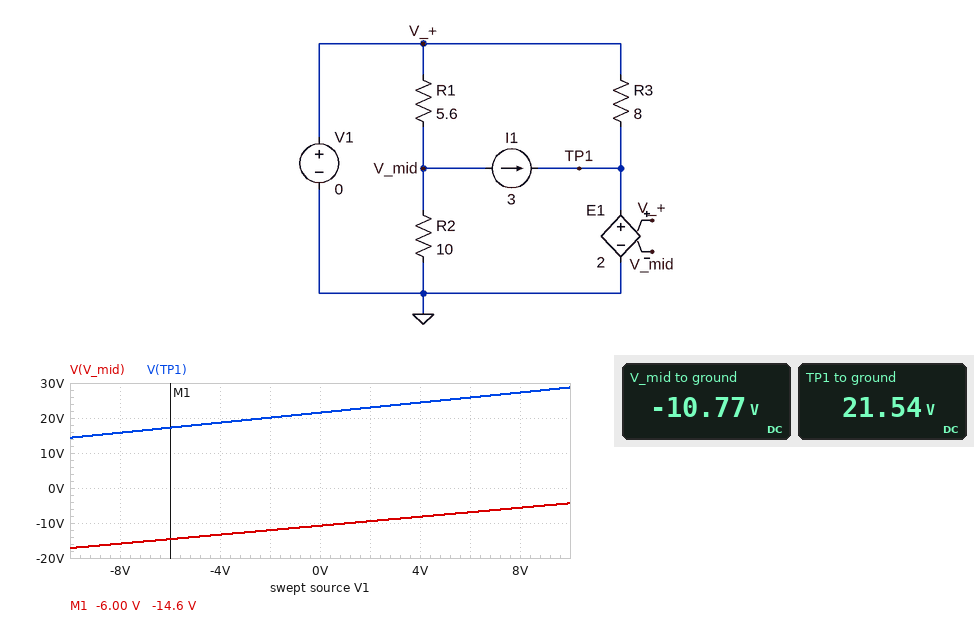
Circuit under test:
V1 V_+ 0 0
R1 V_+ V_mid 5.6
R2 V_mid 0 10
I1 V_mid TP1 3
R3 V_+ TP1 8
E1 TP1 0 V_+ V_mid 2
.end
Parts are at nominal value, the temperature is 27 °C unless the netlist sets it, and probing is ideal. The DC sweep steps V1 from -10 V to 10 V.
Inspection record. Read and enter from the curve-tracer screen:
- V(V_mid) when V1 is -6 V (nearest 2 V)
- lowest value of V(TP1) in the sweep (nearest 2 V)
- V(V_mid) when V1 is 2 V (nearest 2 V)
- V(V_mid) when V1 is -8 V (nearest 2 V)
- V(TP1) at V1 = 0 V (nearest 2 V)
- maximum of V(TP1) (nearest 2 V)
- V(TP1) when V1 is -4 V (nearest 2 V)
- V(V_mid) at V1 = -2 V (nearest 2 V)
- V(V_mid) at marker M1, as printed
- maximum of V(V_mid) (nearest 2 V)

-14 V
14 V
-10 V
-16 V
22 V
28 V
18 V
-12 V
-14.6 V
-4 V
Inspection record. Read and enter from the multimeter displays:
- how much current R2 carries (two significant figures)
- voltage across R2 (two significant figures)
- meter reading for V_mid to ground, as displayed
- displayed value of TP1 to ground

1.1 A
11 V
-10.77 V
21.54 V
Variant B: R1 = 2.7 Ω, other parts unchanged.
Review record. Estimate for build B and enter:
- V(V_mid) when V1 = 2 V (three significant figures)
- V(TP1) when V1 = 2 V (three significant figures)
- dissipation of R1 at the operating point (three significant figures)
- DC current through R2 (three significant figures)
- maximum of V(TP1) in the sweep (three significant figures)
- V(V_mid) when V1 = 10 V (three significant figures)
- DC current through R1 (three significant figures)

-4.80 V
13.6 V
15.1 W
638 mA
17.0 V
1.50 V
2.36 A
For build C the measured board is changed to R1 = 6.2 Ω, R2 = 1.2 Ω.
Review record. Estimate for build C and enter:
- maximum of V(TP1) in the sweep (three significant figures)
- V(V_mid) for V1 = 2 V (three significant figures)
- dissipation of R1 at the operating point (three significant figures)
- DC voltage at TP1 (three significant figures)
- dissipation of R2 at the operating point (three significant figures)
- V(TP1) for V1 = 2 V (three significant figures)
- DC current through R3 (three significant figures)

22.8 V
-2.69 V
1.47 W
6.03 V
7.58 W
9.38 V
754 mA
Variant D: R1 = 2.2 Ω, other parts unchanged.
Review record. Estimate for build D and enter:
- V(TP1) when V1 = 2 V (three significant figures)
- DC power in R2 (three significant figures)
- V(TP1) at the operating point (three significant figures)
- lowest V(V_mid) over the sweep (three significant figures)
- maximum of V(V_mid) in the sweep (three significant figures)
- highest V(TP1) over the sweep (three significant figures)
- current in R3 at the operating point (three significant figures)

11.5 V
2.93 W
10.8 V
-13.6 V
2.79 V
14.4 V
1.35 A
